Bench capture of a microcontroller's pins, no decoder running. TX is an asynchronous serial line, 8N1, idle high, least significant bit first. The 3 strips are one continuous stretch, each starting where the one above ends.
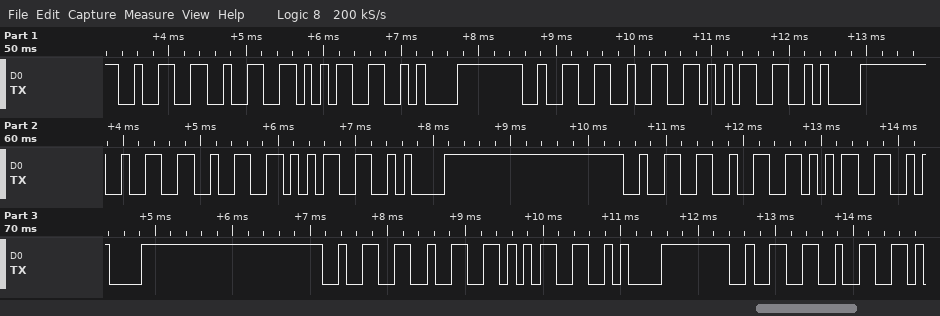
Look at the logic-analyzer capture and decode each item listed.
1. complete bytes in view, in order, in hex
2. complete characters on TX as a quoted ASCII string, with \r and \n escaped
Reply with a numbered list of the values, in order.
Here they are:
1. 32 32 35 0A 32 32 35 0A 32 32 35 0A 32 32 35 0A 32 32 35 0A 32 32
2. "225\n225\n225\n225\n225\n22"
